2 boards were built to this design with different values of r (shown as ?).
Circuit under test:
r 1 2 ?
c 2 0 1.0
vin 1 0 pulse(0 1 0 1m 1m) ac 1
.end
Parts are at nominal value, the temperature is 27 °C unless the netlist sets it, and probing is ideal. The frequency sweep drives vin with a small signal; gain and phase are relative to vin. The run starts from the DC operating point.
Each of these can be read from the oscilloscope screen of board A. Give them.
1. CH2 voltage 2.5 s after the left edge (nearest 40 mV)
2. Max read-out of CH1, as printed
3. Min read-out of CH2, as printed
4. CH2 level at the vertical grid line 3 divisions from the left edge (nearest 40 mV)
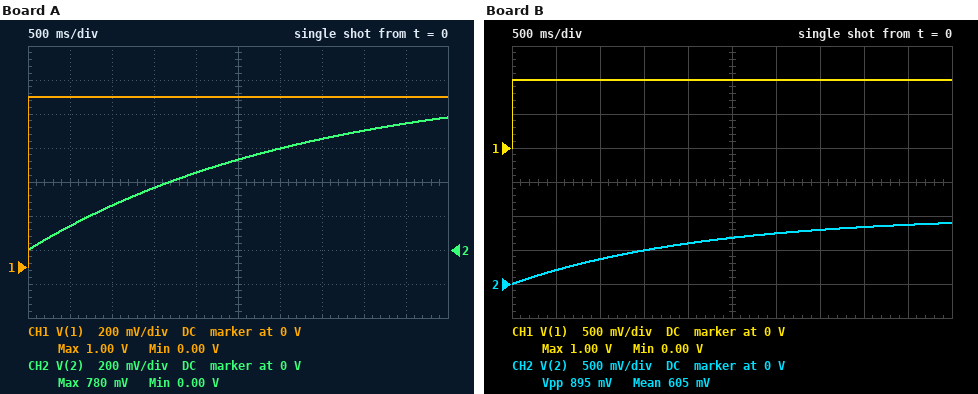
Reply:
520 mV
1.00 V
0.00 V
360 mV
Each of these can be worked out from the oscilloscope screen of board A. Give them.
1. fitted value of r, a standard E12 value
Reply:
3.3 Ω
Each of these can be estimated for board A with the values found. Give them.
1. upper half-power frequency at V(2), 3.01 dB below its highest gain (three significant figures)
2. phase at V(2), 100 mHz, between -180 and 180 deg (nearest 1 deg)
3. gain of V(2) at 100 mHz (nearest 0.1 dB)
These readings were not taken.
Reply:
48.2 mHz
-64 deg
-7.2 dB
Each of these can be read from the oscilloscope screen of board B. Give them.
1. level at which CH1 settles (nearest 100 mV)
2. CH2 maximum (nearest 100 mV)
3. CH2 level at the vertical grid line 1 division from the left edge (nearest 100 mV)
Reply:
1.0 V
900 mV
200 mV
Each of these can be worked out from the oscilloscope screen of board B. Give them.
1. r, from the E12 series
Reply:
2.2 Ω
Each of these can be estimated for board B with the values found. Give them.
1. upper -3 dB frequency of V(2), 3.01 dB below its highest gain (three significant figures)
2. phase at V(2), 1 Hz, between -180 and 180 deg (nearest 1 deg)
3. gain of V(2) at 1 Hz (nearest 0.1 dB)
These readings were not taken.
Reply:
72.3 mHz
-86 deg
-22.8 dB
